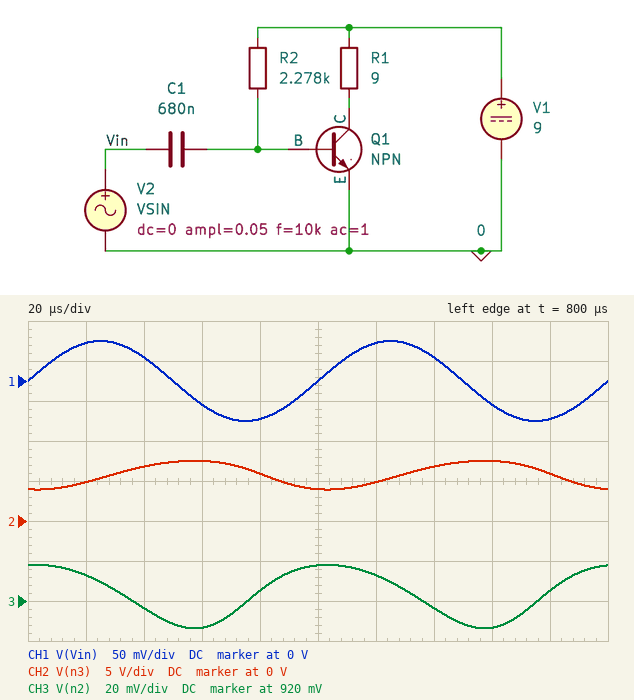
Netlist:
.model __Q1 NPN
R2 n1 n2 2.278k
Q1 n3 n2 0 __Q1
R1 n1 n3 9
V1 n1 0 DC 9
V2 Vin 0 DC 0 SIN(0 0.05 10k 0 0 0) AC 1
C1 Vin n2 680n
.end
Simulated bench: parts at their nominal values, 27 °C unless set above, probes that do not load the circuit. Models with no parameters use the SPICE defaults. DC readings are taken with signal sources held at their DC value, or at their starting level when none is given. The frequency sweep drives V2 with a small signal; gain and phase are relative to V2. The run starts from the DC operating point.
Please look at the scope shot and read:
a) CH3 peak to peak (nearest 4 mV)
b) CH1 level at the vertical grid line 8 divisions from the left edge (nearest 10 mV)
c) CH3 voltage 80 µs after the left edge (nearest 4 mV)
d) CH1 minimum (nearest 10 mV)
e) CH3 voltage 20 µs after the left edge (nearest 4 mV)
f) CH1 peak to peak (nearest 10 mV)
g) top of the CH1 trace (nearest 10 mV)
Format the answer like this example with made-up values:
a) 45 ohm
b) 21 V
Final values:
a) 32 mV
b) -30 mV
c) 924 mV
d) -50 mV
e) 932 mV
f) 100 mV
g) 50 mV
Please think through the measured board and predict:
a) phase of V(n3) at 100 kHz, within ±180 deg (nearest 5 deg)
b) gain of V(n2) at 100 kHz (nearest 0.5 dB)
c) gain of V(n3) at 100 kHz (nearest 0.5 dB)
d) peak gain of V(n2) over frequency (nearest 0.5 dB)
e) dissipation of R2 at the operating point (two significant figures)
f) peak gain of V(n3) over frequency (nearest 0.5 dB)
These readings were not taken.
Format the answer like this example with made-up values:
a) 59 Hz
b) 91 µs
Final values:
a) -160 deg
b) -0.5 dB
c) 41.5 dB
d) 0 dB
e) 29 mW
f) 42.0 dB
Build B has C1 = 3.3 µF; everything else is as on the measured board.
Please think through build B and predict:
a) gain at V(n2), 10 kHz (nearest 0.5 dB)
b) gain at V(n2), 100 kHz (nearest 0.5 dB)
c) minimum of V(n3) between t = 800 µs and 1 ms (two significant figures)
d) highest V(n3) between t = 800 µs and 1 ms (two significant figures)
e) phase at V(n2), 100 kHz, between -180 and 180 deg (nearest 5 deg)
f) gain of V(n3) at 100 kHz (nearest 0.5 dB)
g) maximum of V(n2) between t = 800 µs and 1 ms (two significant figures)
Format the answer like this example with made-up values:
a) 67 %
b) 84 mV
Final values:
a) -1.5 dB
b) 0 dB
c) 180 mV
d) 8.7 V
e) 5 deg
f) 42.0 dB
g) 950 mV
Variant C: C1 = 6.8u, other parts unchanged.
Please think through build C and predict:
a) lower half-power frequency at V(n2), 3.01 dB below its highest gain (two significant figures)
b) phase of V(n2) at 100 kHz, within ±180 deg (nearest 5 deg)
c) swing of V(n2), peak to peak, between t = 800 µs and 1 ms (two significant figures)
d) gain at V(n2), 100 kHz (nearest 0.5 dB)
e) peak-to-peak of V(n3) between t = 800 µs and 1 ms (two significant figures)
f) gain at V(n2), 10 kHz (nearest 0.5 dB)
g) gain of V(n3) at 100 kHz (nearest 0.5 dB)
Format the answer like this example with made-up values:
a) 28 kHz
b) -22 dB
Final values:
a) 3.2 kHz
b) 0 deg
c) 95 mV
d) 0 dB
e) 8.6 V
f) -0.5 dB
g) 42.0 dB
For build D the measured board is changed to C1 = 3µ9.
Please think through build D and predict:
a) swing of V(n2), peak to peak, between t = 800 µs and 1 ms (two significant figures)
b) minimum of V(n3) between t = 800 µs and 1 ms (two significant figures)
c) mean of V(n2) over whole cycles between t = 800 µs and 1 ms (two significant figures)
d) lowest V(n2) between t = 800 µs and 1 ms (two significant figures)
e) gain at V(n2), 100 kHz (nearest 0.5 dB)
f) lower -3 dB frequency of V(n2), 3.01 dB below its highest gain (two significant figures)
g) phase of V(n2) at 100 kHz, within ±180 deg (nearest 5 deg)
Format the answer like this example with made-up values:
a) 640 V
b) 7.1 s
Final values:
a) 90 mV
b) 160 mV
c) 910 mV
d) 860 mV
e) 0 dB
f) 5.6 kHz
g) 5 deg
